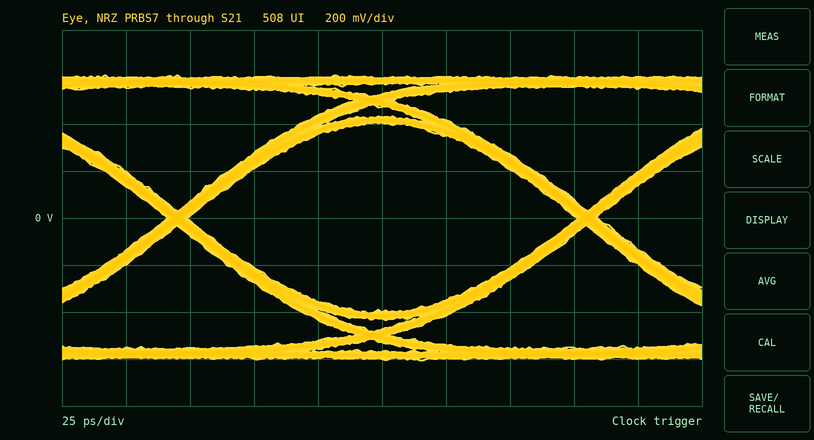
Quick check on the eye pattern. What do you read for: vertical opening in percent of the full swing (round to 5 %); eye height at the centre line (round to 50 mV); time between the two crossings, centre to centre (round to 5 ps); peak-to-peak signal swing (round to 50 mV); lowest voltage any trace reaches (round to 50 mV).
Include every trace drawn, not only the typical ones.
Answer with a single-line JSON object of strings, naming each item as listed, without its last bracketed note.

{"vertical opening in percent of the full swing": "65 %", "eye height at the centre line": "800 mV", "time between the two crossings, centre to centre": "160 ps", "peak-to-peak signal swing": "1.20 V", "lowest voltage any trace reaches": "-600 mV"}
